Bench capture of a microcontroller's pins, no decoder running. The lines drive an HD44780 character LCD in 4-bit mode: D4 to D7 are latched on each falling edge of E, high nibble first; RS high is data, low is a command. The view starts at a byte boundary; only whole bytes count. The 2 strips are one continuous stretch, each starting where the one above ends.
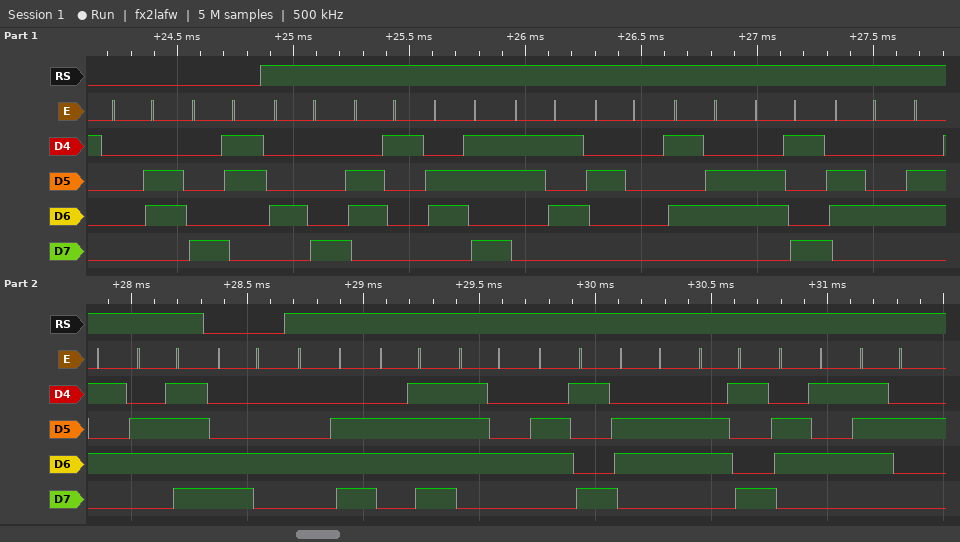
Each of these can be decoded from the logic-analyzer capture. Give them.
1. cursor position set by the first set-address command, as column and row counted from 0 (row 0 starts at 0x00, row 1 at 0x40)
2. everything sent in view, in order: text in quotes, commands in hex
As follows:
column 3, row 0
0x06 0x83 "Hak5 Video" 0xC4 "Notifier"
